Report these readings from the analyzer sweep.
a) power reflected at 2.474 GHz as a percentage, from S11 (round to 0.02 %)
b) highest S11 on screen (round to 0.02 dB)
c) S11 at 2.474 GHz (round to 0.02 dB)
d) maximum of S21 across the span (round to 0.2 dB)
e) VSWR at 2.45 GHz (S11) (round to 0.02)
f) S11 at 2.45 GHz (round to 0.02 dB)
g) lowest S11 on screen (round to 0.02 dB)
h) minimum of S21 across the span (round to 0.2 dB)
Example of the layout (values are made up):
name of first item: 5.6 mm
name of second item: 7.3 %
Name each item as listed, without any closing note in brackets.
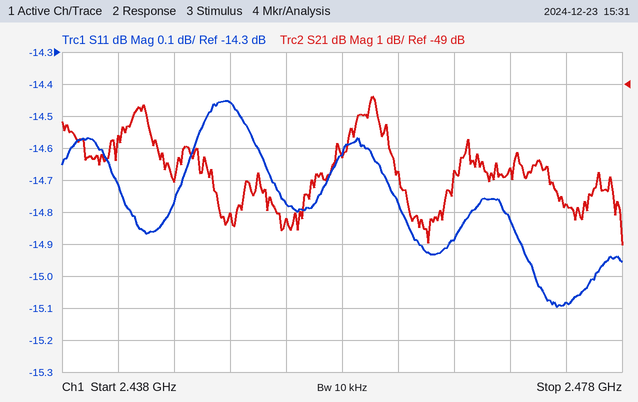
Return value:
power reflected at 2.474 GHz as a percentage, from S11: 3.10 %
highest S11 on screen: -14.46 dB
S11 at 2.474 GHz: -15.08 dB
maximum of S21 across the span: -49.4 dB
VSWR at 2.45 GHz (S11): 1.46
S11 at 2.45 GHz: -14.46 dB
lowest S11 on screen: -15.10 dB
minimum of S21 across the span: -54.0 dB
